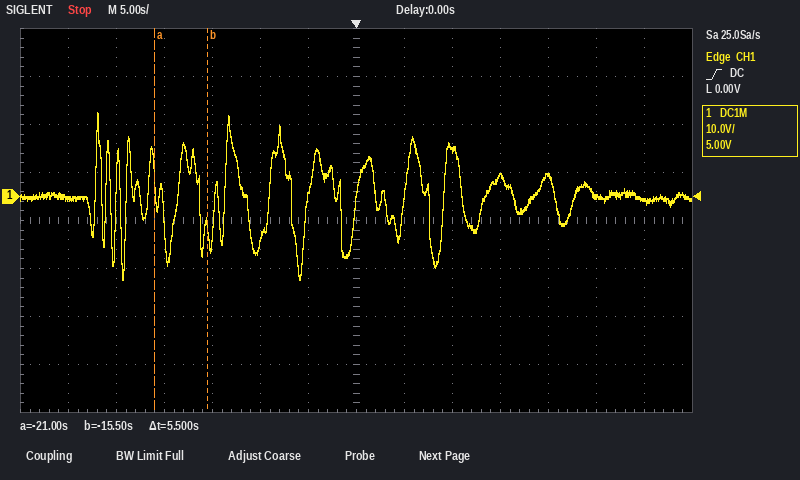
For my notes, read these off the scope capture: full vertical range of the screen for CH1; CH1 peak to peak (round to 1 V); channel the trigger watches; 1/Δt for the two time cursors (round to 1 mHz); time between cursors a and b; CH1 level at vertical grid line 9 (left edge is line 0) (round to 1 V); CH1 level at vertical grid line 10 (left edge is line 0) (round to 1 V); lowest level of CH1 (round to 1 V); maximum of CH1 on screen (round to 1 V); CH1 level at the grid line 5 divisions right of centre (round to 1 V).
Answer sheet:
80 V
35 V
CH1
182 mHz
5.5 s
10 V
4 V
-17 V
18 V
0 V
